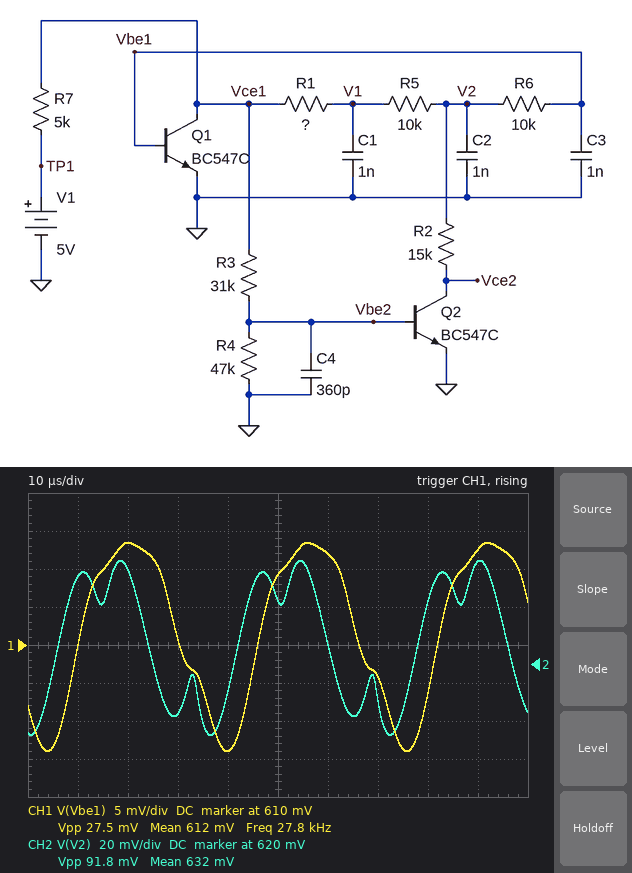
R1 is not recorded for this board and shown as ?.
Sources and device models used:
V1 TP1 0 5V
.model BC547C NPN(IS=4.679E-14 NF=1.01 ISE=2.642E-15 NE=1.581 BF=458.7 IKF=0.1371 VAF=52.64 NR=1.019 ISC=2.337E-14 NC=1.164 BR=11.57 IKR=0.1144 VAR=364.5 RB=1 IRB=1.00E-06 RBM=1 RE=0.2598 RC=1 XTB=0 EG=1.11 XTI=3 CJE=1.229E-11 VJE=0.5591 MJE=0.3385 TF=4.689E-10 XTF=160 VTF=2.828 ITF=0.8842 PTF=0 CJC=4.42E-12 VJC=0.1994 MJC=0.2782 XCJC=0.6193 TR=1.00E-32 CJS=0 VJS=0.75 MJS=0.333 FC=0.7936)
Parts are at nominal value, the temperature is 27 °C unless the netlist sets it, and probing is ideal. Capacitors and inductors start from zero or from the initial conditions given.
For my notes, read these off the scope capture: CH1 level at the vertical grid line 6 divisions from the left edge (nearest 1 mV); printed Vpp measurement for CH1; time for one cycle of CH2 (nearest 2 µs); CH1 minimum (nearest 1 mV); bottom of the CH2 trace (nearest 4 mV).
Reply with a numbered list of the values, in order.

1. 622 mV
2. 27.5 mV
3. 36 µs
4. 596 mV
5. 584 mV
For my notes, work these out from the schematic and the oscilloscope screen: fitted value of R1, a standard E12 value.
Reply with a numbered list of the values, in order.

1. 12 kΩ
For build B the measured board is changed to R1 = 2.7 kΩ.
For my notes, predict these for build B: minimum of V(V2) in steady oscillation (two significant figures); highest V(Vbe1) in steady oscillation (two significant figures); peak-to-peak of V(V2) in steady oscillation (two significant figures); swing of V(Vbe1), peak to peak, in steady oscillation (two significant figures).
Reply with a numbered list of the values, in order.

1. 570 mV
2. 620 mV
3. 110 mV
4. 20 mV
